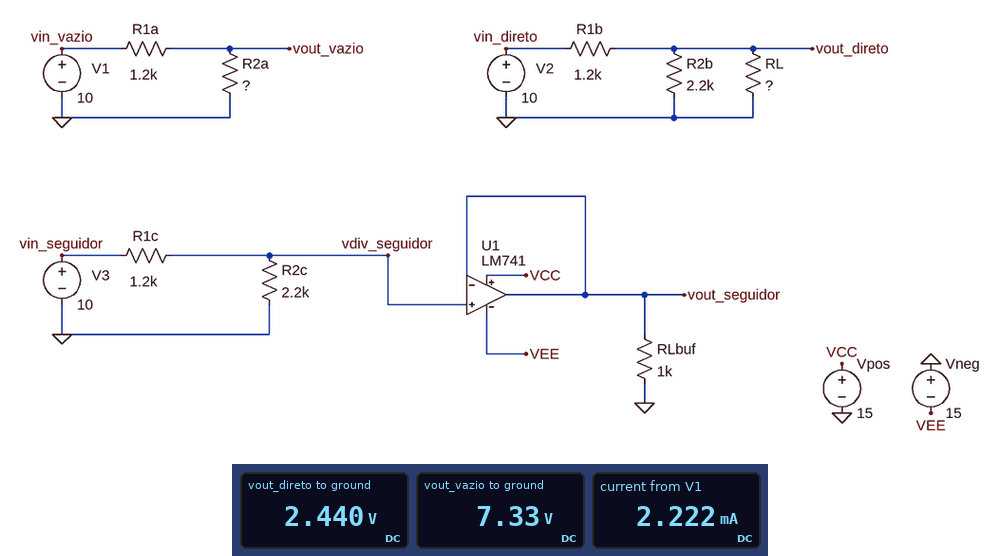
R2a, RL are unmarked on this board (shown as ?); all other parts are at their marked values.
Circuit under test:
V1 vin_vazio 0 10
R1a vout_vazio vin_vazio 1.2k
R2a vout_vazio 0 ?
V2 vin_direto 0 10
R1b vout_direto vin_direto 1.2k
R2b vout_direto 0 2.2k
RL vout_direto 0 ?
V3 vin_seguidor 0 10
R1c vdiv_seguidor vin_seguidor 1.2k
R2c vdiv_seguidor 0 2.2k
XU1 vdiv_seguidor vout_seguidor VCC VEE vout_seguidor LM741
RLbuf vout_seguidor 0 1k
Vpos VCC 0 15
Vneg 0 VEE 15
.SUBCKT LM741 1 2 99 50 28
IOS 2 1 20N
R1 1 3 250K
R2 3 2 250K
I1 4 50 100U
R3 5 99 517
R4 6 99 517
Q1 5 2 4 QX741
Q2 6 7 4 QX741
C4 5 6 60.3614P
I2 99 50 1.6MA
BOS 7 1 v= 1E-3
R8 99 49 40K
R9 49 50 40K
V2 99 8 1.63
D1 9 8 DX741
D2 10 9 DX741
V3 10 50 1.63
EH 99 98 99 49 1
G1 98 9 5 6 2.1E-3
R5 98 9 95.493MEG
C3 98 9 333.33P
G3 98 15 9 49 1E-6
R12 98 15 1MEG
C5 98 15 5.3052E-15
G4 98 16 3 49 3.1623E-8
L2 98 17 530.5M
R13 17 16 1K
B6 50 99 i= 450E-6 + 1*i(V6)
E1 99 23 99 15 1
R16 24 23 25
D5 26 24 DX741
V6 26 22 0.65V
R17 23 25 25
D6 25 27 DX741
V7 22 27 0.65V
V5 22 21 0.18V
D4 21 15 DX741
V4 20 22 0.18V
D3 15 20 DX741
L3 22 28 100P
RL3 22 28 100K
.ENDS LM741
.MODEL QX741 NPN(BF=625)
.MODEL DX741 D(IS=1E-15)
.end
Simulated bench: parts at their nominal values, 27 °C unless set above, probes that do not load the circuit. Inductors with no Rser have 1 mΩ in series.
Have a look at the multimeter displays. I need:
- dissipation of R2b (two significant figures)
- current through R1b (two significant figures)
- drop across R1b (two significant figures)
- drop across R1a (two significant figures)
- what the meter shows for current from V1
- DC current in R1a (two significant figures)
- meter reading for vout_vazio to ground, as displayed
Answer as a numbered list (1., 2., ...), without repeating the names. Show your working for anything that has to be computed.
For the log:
1. (2.44 V)^2 / 2.2 kΩ = 2.7 mW
2. (10 V - 2.44 V) / 1.2 kΩ = 6.3 mA
3. 10 V - 2.44 V = 7.6 V
4. 10 V - 7.33 V = 2.7 V
5. 2.222 mA
6. (10 V - 7.33 V) / 1.2 kΩ = 2.2 mA
7. 7.33 V
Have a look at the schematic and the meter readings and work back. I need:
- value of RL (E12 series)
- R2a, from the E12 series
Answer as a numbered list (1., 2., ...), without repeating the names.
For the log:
1. 470 Ω
2. 3.3 kΩ
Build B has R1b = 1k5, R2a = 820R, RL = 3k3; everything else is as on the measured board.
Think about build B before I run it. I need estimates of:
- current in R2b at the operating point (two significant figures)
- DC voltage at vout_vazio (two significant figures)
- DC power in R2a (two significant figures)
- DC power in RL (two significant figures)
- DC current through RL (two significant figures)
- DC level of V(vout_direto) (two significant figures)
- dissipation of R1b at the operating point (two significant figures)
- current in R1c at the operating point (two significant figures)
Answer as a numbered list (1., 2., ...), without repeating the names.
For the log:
1. 2.1 mA
2. 4.1 V
3. 20 mW
4. 6.6 mW
5. 1.4 mA
6. 4.7 V
7. 19 mW
8. 2.9 mA
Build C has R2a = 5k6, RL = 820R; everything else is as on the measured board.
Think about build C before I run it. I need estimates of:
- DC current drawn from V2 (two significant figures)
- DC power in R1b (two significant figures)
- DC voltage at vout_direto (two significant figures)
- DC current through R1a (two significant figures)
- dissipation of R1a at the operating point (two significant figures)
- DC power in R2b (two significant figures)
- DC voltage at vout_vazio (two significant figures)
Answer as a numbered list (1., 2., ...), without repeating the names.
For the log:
1. 5.6 mA
2. 37 mW
3. 3.3 V
4. 1.5 mA
5. 2.6 mW
6. 5.0 mW
7. 8.2 V
